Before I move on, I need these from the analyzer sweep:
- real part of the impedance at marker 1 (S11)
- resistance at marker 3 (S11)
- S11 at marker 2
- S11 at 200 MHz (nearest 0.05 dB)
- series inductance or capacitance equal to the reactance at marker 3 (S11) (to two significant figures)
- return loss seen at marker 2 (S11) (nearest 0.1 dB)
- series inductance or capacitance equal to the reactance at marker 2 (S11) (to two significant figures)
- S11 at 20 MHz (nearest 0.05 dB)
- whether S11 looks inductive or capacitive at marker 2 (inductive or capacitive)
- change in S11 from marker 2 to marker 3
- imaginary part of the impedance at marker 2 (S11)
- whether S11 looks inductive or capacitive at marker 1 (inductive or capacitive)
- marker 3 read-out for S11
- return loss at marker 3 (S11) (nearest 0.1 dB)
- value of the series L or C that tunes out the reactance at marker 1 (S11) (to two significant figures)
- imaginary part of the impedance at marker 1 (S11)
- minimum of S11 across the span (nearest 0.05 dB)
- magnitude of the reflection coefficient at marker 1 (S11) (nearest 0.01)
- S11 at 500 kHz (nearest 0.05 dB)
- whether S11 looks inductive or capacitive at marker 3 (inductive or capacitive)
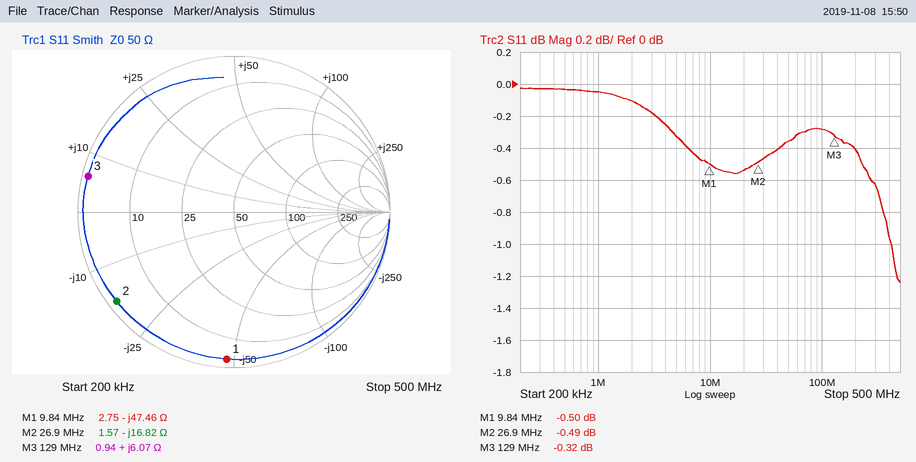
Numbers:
2.75 Ω
0.94 Ω
-0.49 dB
-0.40 dB
7.5 nH
0.5 dB
350 pF
-0.55 dB
capacitive
0.17 dB
-16.82 Ω
capacitive
-0.32 dB
0.3 dB
770 nH
-47.46 Ω
-1.25 dB
0.94
-0.05 dB
inductive
